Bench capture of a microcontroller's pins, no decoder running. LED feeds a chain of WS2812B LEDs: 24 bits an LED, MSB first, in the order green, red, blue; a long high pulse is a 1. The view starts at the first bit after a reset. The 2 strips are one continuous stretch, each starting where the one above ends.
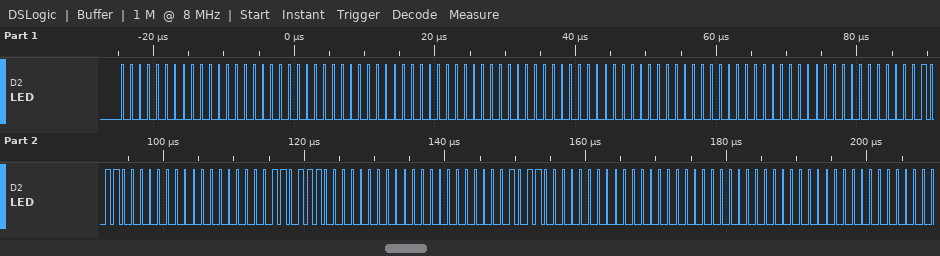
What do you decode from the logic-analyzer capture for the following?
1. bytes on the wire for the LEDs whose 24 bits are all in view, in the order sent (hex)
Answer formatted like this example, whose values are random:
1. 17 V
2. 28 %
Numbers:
1. 00 00 00 00 00 00 00 00 00 00 00 16 00 00 DC 00 00 16 00 00 00
